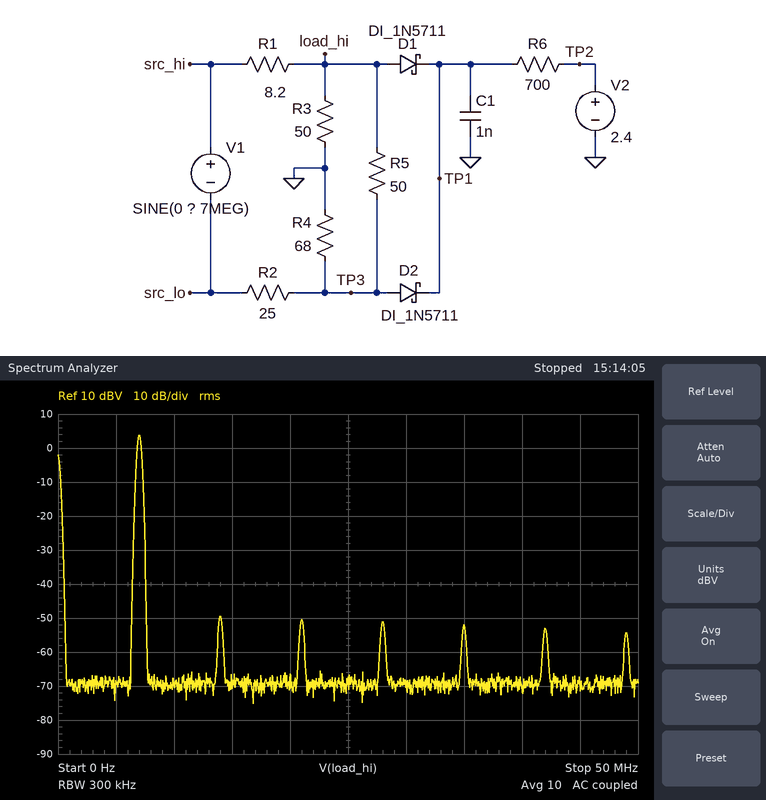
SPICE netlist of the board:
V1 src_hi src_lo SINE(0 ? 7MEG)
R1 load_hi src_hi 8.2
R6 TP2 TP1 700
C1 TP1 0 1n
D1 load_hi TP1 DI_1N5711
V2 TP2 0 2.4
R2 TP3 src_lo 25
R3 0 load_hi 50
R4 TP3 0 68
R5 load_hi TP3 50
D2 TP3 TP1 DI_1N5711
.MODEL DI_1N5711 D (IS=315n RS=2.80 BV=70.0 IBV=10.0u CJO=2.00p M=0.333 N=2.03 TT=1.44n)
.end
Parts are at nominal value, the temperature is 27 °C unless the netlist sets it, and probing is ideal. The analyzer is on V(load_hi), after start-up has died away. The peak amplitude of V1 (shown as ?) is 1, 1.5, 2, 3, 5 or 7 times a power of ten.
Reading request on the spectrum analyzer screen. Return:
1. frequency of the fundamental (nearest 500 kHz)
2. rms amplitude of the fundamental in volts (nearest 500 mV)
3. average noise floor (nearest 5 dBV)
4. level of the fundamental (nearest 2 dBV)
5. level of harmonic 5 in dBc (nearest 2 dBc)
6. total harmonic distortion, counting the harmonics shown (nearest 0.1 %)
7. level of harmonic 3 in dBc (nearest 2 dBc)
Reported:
7.0 MHz
1.5 V
-70 dBV
4 dBV
-56 dBc
0.4 %
-54 dBc
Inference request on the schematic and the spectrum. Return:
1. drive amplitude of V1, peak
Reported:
10 V
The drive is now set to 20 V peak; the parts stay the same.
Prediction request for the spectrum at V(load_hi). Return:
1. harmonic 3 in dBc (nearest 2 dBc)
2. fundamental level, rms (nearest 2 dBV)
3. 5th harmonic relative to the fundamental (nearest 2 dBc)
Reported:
-32 dBc
10 dBV
-38 dBc
